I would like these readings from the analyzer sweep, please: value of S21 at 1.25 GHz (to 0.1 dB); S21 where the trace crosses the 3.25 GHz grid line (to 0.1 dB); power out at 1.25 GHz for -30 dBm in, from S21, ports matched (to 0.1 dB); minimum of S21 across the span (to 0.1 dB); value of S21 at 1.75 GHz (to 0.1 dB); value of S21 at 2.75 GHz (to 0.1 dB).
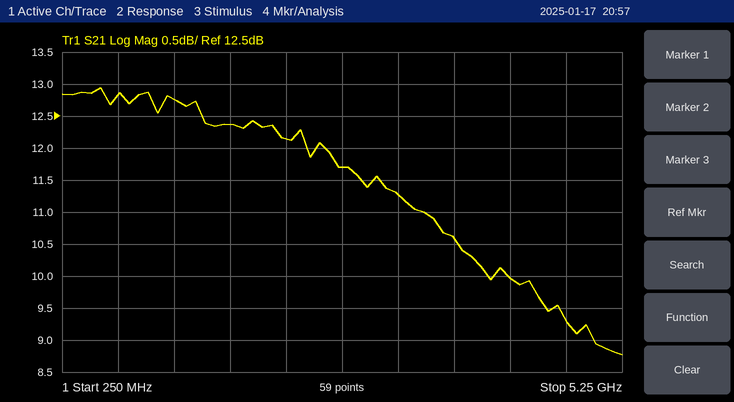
12.8 dB
11.3 dB
-17.2 dBm
8.8 dB
12.4 dB
11.7 dB
